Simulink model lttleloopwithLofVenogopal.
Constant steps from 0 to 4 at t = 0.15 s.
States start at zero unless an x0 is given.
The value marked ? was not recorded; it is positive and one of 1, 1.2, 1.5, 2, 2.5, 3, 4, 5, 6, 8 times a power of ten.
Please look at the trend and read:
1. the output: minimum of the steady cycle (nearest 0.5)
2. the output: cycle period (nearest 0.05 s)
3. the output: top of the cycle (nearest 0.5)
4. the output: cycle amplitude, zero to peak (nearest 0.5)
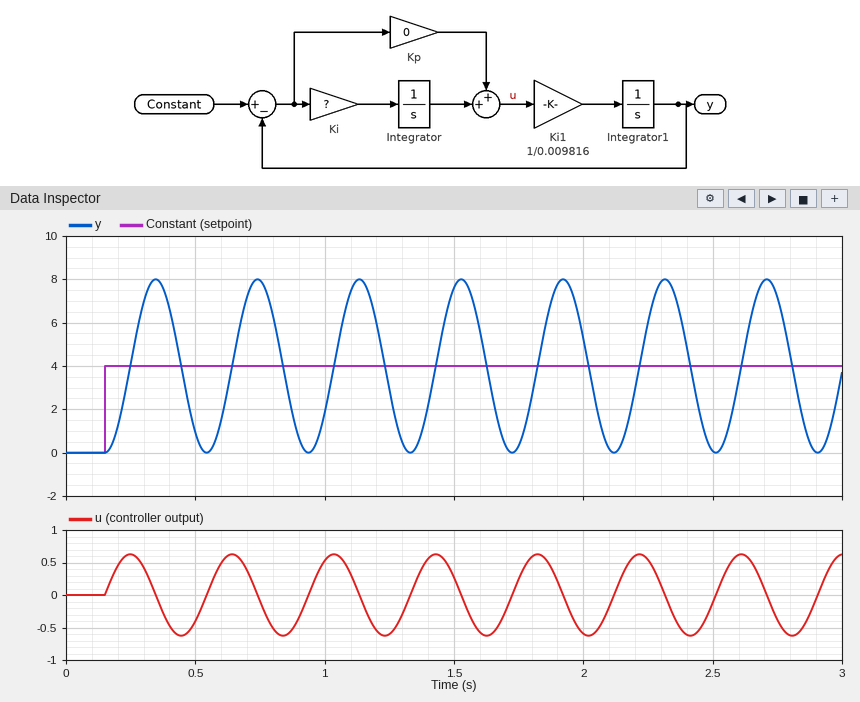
0.0
0.40 s
8.0
4.0
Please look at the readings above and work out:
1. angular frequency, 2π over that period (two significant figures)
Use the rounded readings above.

16 rad/s
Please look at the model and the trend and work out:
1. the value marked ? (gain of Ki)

2.5
